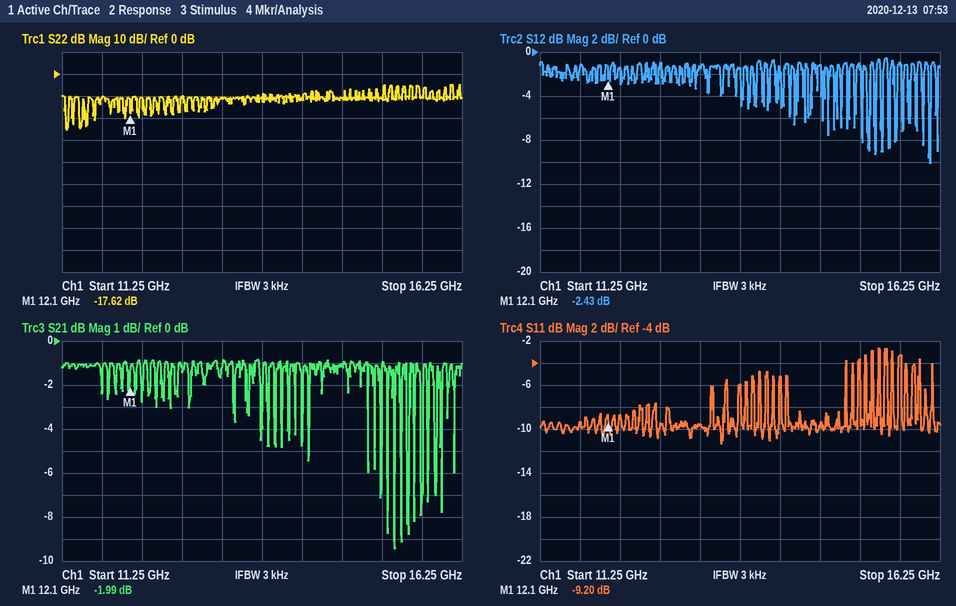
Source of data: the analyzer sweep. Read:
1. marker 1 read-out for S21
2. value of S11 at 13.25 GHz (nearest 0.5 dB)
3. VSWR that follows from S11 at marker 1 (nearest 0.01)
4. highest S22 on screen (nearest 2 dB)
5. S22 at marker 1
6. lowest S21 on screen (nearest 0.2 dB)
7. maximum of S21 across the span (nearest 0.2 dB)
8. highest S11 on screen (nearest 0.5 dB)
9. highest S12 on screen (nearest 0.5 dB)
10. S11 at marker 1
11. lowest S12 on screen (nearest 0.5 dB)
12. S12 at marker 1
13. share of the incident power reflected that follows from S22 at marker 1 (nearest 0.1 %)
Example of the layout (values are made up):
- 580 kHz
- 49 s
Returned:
- -1.99 dB
- -9.5 dB
- 2.06
- -4 dB
- -17.62 dB
- -9.4 dB
- -0.8 dB
- -2.5 dB
- -0.5 dB
- -9.20 dB
- -10.0 dB
- -2.43 dB
- 1.7 %
